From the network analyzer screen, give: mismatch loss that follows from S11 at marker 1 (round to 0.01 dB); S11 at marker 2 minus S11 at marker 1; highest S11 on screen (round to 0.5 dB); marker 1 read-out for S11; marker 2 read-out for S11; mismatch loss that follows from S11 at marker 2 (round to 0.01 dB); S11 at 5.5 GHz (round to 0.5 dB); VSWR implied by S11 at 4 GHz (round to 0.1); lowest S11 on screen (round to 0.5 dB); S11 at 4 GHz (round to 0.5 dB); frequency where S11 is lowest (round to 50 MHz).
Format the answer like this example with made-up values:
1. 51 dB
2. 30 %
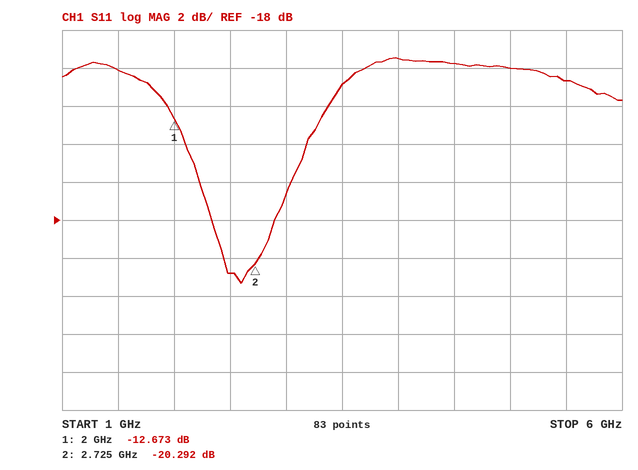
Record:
1. 0.24 dB
2. -7.619 dB
3. -9.5 dB
4. -12.673 dB
5. -20.292 dB
6. 0.04 dB
7. -10.5 dB
8. 2.0
9. -21.5 dB
10. -9.5 dB
11. 2.60 GHz
